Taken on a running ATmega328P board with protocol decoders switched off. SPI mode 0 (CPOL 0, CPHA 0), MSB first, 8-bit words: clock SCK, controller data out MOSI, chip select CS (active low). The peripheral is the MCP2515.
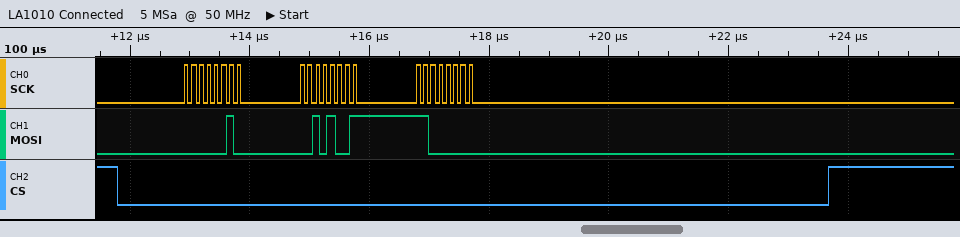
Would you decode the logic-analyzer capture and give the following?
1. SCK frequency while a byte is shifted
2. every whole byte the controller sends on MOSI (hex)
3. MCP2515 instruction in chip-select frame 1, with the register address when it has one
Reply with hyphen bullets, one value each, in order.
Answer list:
- 8 MHz
- 02 29 C0
- WRITE 0x29
